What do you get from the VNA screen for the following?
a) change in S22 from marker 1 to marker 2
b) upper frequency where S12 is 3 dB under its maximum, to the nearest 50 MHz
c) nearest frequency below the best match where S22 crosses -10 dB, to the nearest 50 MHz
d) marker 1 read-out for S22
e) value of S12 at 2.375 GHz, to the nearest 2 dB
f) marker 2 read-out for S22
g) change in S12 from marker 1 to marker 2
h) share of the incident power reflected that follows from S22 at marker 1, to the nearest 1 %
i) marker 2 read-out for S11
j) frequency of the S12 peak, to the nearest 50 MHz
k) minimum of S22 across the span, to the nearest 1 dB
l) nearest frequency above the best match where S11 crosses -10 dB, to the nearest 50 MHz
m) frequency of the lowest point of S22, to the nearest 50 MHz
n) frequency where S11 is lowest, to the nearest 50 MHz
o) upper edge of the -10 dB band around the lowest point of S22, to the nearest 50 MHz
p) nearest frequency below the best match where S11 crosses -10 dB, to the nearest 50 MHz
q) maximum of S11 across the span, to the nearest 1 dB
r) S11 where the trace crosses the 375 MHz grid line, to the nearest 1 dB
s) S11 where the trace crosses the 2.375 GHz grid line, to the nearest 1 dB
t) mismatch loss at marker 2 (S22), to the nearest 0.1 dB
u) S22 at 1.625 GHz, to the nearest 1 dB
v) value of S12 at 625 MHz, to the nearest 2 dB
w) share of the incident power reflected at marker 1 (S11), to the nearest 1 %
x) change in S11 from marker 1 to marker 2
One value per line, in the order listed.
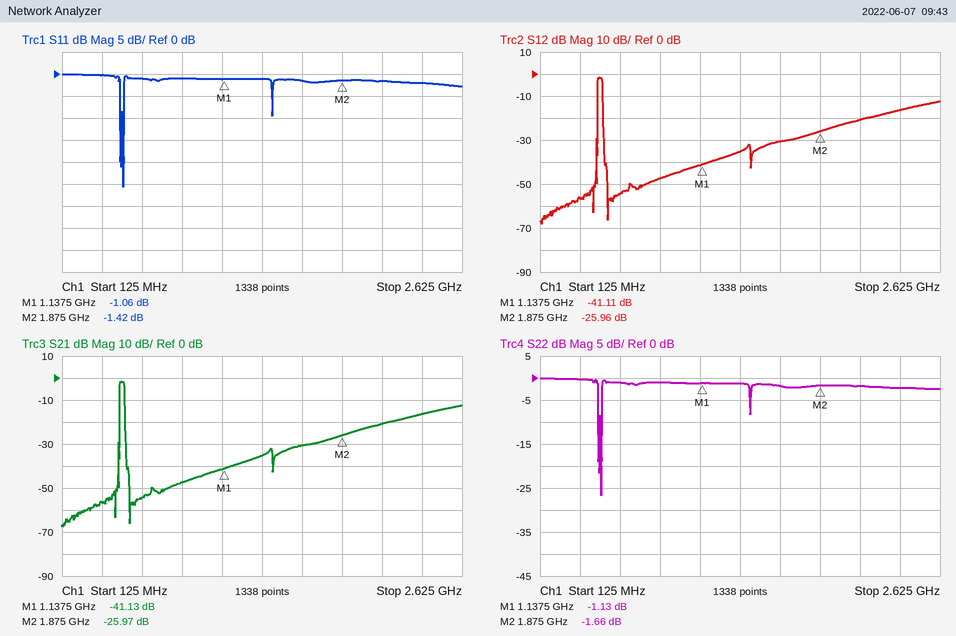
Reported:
-0.53 dB
500 MHz
500 MHz
-1.13 dB
-16 dB
-1.66 dB
15.15 dB
77 %
-1.42 dB
500 MHz
-27 dB
500 MHz
500 MHz
500 MHz
500 MHz
500 MHz
0 dB
0 dB
-2 dB
5.0 dB
-2 dB
-54 dB
78 %
-0.36 dB
